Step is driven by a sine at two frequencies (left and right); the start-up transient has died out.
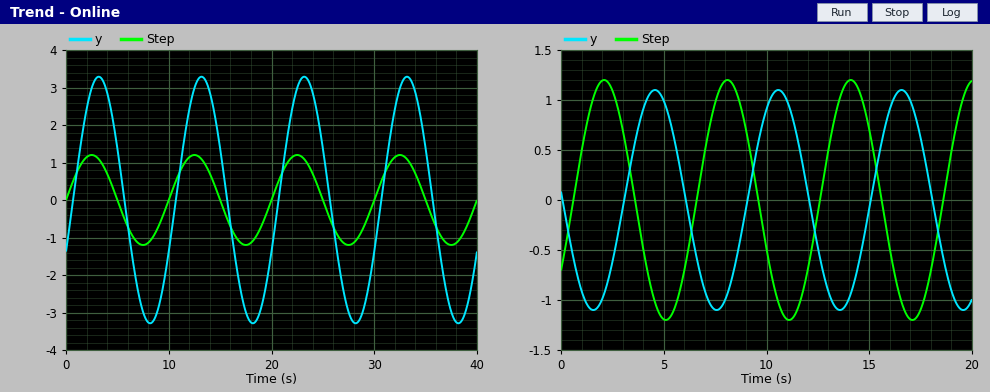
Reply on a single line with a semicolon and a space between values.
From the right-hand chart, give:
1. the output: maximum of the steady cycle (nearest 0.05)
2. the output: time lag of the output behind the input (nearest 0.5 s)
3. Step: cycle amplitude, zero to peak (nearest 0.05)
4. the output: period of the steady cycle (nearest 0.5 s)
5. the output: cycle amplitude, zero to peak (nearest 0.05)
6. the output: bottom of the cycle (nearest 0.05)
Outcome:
1.10; 2.5 s; 1.20; 6.0 s; 1.10; -1.10
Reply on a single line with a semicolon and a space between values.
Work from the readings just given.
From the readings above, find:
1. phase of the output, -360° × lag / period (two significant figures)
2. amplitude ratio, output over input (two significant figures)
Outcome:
-150°; 0.92
